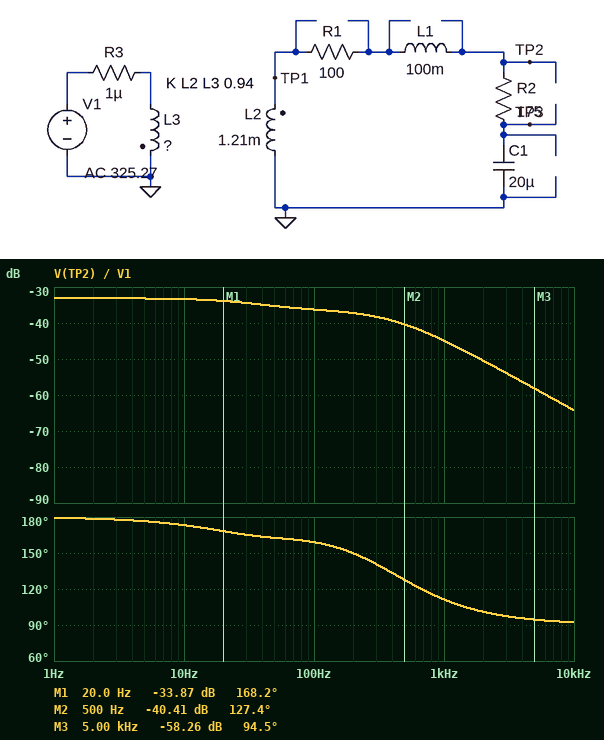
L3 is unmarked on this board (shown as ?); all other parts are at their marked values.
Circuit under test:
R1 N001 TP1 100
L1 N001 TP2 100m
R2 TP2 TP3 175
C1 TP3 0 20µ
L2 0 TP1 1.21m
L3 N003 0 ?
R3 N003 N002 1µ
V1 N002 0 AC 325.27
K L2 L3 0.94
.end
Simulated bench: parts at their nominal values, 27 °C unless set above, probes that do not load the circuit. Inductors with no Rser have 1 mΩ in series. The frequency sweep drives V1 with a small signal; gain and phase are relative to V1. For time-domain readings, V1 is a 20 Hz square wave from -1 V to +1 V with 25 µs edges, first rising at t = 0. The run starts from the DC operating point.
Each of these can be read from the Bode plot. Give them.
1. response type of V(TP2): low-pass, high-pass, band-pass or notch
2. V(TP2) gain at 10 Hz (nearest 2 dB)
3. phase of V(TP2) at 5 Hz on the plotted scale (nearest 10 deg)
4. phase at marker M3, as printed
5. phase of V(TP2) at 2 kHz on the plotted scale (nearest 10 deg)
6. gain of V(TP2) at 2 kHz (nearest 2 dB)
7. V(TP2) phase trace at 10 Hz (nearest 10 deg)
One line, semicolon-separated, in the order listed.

low-pass; -34 dB; 180 deg; 94.5 deg; 100 deg; -50 dB; 170 deg
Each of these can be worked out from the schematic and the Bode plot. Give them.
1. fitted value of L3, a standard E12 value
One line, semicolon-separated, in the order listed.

2.2 H
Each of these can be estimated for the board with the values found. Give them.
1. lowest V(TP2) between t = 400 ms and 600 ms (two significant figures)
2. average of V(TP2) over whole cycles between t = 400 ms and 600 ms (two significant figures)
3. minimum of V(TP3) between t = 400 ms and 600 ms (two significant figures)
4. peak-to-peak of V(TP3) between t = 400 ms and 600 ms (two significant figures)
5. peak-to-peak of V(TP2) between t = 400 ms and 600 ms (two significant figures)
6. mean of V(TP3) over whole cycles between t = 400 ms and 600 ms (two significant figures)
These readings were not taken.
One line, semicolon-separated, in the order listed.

-44 mV; -22 mV; -44 mV; 43 mV; 44 mV; -22 mV
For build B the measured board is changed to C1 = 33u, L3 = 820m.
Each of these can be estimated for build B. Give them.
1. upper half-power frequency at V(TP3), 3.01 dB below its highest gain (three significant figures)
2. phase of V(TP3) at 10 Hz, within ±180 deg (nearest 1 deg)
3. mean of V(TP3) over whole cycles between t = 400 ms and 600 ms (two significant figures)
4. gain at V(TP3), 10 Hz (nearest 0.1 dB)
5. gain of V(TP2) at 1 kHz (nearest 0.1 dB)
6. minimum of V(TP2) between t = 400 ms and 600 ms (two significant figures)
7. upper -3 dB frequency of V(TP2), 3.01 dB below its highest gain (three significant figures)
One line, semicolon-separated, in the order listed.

18.3 Hz; 150 deg; -36 mV; -30.0 dB; -40.7 dB; -71 mV; 50.0 Hz
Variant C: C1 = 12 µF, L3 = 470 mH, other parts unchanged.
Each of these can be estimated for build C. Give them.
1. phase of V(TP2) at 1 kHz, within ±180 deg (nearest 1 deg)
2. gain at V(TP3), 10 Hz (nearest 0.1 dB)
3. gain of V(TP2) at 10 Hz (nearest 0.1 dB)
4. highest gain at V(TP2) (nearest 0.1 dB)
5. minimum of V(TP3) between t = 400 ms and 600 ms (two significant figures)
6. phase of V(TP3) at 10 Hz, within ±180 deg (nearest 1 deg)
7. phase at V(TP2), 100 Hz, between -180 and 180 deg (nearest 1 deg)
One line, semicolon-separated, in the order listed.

110 deg; -26.6 dB; -26.5 dB; -26.4 dB; -95 mV; 168 deg; 157 deg
